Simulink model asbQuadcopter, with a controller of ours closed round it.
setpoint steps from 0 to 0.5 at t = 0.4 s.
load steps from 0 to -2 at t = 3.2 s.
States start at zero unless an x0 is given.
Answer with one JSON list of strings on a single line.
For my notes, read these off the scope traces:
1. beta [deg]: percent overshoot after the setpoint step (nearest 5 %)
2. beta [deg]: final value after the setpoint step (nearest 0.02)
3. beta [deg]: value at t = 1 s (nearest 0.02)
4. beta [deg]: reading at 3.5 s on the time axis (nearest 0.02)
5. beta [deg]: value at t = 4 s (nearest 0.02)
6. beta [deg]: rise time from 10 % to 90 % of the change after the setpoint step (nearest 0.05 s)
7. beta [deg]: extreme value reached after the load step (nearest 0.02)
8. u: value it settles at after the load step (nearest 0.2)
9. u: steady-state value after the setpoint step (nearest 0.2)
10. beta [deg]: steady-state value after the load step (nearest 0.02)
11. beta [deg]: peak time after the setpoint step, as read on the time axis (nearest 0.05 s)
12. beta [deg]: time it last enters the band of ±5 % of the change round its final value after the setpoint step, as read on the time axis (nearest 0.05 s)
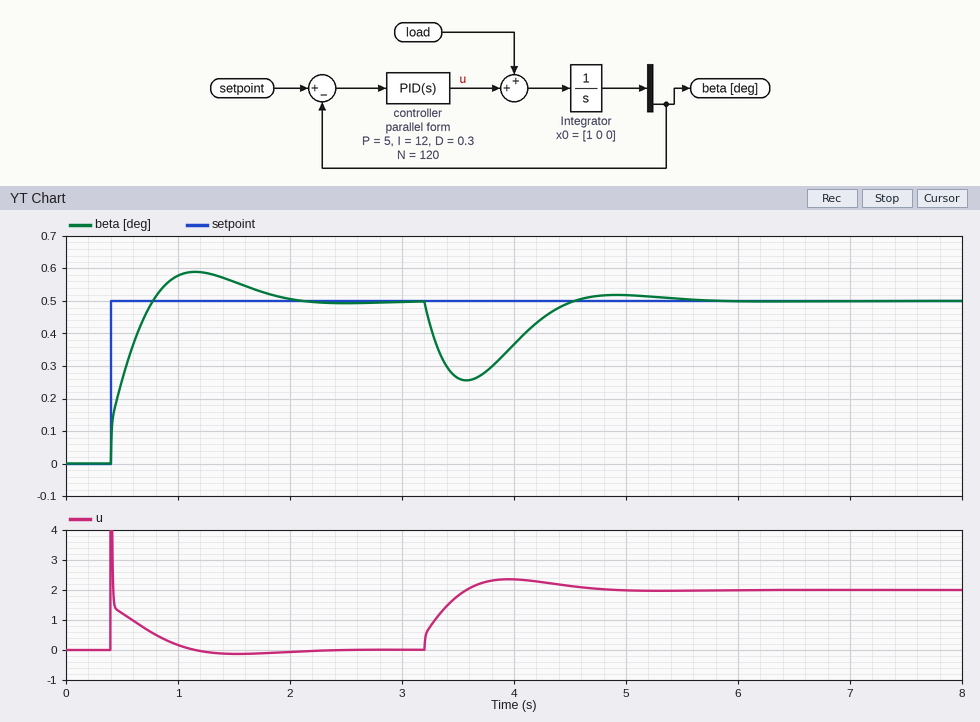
["20 %", "0.50", "0.58", "0.26", "0.36", "0.30 s", "0.26", "2.0", "0.0", "0.50", "1.15 s", "1.80 s"]
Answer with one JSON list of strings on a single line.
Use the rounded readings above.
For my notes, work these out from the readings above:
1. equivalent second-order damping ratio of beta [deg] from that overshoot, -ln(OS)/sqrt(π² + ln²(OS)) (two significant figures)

["0.46"]
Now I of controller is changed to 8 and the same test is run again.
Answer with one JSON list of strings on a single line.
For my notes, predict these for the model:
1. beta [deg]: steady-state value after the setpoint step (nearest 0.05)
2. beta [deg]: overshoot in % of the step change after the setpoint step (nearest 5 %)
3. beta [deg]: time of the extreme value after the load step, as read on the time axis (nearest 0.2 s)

["0.50", "15 %", "3.6 s"]
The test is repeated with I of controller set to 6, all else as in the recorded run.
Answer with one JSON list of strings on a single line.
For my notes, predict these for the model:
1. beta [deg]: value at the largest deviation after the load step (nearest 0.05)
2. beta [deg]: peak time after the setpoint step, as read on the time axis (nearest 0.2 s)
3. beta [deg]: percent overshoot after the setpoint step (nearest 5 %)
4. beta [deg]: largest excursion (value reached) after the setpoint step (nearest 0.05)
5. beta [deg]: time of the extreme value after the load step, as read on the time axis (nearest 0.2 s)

["0.20", "1.4 s", "10 %", "0.55", "3.6 s"]
